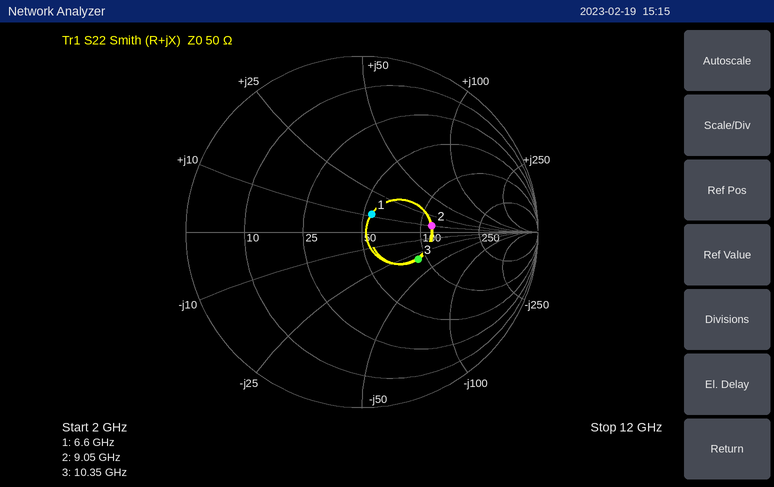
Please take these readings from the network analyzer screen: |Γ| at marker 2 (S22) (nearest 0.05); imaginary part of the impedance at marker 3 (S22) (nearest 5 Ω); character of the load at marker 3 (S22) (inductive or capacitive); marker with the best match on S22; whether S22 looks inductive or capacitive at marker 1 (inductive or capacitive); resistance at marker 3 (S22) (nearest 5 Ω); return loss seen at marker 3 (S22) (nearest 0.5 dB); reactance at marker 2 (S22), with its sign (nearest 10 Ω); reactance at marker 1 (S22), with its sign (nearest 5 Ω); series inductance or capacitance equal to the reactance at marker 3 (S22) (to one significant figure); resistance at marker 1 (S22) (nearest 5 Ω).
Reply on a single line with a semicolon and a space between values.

0.40; -30 Ω; capacitive; marker 1; inductive; 90 Ω; 9.0 dB; +10 Ω; +10 Ω; 500 fF; 55 Ω
